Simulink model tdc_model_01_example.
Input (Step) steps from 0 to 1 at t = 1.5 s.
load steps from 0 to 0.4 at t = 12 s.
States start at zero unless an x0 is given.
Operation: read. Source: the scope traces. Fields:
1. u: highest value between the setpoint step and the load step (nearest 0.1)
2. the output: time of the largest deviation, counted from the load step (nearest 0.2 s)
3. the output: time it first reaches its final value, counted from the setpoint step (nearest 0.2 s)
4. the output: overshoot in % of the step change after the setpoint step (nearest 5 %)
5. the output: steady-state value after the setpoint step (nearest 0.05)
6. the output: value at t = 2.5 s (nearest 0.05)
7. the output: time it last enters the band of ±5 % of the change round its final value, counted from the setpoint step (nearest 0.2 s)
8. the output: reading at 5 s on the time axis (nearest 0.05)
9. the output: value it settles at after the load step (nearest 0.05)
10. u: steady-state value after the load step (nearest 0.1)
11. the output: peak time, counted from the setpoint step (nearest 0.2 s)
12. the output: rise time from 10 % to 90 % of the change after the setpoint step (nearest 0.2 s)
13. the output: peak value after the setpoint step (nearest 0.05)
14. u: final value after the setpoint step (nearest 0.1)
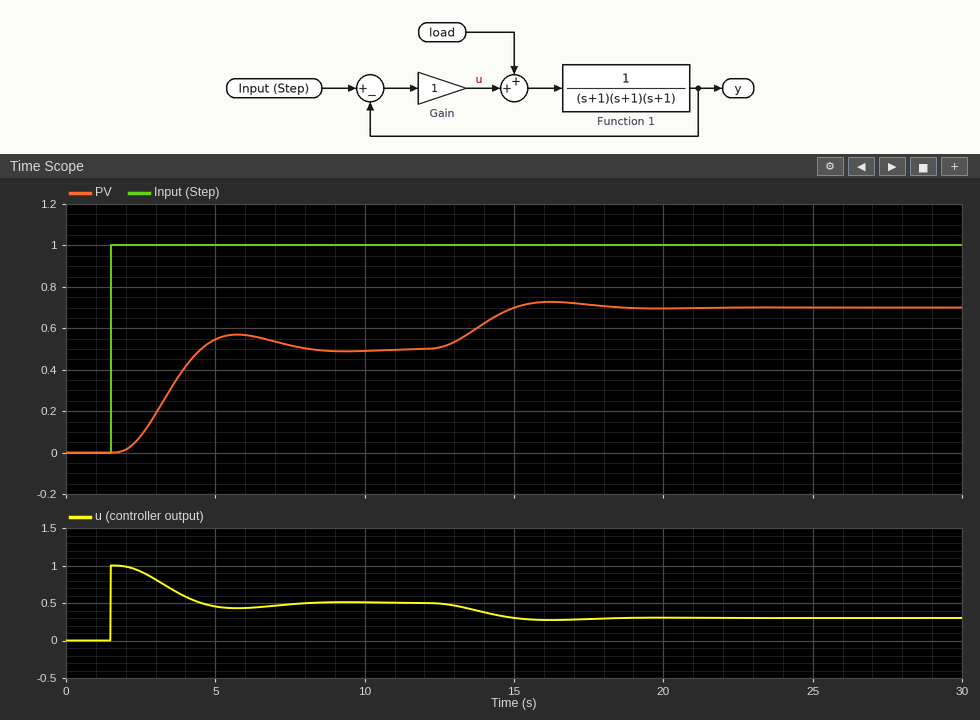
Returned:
1.0
4.2 s
3.0 s
15 %
0.50
0.10
5.8 s
0.55
0.70
0.3
4.2 s
1.8 s
0.55
0.5
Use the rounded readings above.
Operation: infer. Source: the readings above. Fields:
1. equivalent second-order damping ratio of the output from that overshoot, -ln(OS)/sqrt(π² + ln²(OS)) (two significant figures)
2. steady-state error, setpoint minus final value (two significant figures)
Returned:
0.52
0.50
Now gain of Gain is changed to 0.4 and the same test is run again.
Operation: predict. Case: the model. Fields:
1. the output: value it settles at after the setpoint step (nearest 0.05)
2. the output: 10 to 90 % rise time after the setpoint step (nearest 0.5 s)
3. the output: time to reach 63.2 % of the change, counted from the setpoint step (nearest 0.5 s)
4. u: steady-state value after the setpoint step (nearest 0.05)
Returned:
0.30
2.5 s
2.5 s
0.30
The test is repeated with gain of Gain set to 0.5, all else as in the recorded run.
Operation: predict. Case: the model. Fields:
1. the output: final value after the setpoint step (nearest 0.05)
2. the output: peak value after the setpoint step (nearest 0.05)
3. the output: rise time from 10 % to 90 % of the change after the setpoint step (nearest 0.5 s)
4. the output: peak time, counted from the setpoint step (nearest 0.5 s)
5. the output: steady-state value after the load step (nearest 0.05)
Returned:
0.35
0.35
2.5 s
5.5 s
0.60
